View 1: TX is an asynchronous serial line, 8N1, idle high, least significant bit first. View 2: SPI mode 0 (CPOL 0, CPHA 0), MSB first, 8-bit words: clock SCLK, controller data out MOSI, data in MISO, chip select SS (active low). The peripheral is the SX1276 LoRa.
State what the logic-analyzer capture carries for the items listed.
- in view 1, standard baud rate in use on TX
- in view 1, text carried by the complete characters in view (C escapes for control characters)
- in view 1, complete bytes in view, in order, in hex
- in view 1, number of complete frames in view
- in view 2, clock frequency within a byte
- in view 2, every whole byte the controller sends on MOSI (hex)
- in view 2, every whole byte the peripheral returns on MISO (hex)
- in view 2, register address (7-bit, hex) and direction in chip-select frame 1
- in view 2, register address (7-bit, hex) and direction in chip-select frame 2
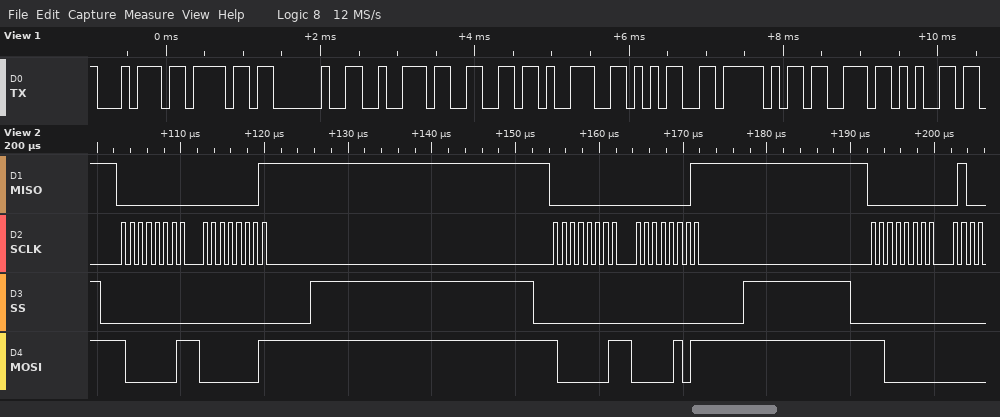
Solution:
9600 baud
"to rf95_se"
74 6F 20 72 66 39 35 5F 73 65
10
1 MHz
81 01 81 05 C0
00 01 00 01 00
0x01 write
0x01 write
